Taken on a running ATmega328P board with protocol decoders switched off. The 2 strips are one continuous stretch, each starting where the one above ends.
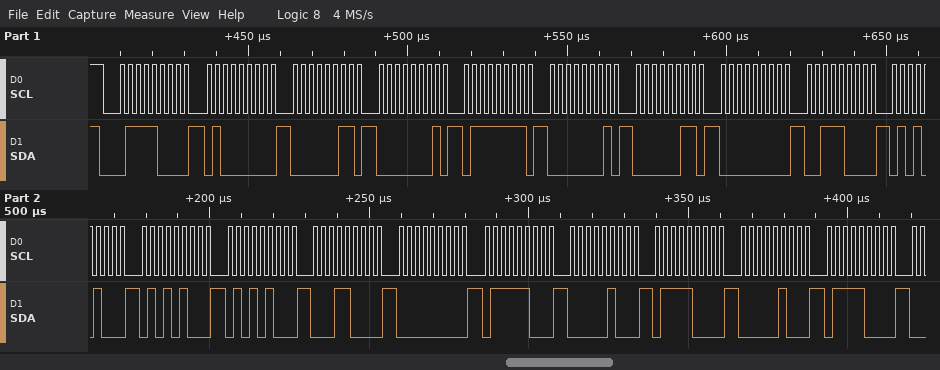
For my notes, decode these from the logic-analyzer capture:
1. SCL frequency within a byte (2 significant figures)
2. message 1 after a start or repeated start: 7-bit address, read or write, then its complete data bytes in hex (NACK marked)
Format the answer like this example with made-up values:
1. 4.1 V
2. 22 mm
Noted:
1. 400 kHz
2. 0x3C write: 40 03 01 7F 01 03 00 38 54 54 54 18 00 7C 04 78 04 78
